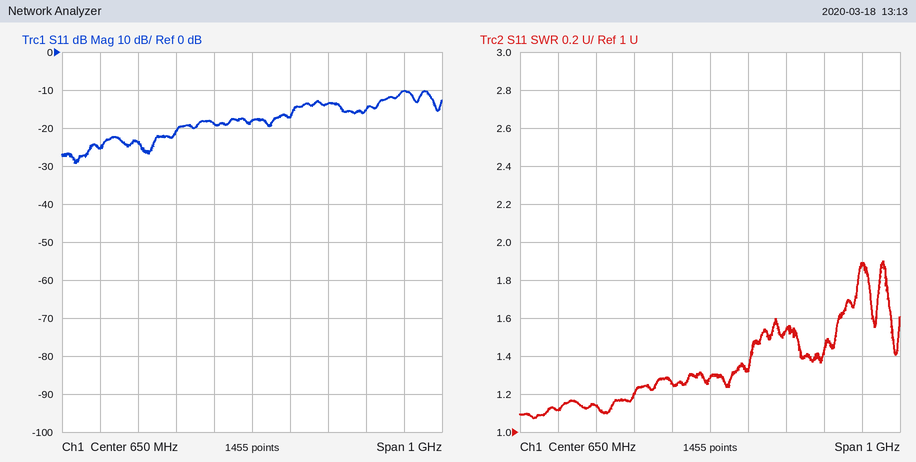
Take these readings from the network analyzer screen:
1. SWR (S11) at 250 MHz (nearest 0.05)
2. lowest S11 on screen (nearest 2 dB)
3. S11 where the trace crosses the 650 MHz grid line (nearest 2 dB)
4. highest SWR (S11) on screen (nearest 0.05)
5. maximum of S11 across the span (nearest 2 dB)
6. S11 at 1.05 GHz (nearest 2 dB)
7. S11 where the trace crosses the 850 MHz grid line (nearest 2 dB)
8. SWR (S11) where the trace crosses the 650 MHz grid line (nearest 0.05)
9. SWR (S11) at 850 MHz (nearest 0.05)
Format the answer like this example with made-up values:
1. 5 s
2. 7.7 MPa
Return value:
1. 1.10
2. -30 dB
3. -18 dB
4. 1.90
5. -10 dB
6. -10 dB
7. -14 dB
8. 1.30
9. 1.55
